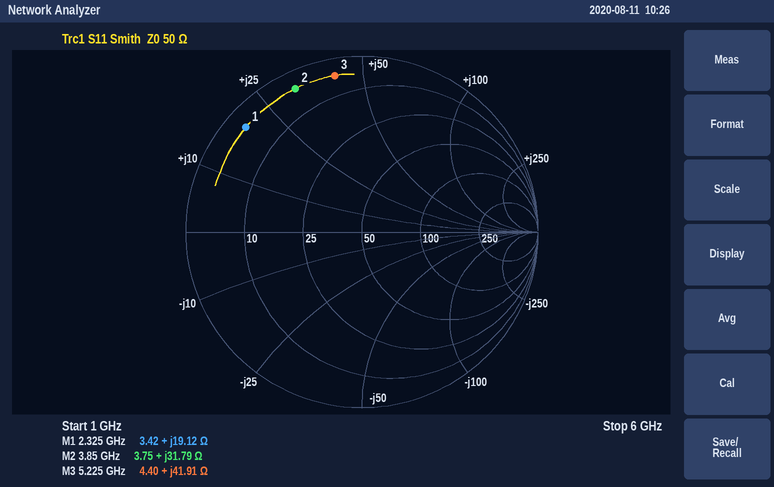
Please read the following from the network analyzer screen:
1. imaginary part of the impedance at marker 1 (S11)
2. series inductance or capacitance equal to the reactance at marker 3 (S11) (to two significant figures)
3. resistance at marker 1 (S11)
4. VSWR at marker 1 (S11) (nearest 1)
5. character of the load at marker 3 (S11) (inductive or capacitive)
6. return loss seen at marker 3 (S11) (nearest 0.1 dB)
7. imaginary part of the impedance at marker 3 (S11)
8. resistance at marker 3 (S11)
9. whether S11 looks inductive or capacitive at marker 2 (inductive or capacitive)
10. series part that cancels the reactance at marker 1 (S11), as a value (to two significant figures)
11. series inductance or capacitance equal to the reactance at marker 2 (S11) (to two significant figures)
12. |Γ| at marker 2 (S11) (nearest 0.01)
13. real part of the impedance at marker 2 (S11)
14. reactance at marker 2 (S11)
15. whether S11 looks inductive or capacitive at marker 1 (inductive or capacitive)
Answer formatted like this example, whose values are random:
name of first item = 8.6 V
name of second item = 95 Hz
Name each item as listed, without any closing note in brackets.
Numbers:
imaginary part of the impedance at marker 1 = +19.12 Ω
series inductance or capacitance equal to the reactance at marker 3 (S11) = 1.3 nH
resistance at marker 1 = 3.42 Ω
VSWR at marker 1 (S11) = 17
character of the load at marker 3 (S11) = inductive
return loss seen at marker 3 (S11) = 0.9 dB
imaginary part of the impedance at marker 3 = +41.91 Ω
resistance at marker 3 = 4.40 Ω
whether S11 looks inductive or capacitive at marker 2 = inductive
series part that cancels the reactance at marker 1 (S11), as a value = 3.6 pF
series inductance or capacitance equal to the reactance at marker 2 (S11) = 1.3 nH
|Γ| at marker 2 (S11) = 0.90
real part of the impedance at marker 2 = 3.75 Ω
reactance at marker 2 = +31.79 Ω
whether S11 looks inductive or capacitive at marker 1 = inductive
